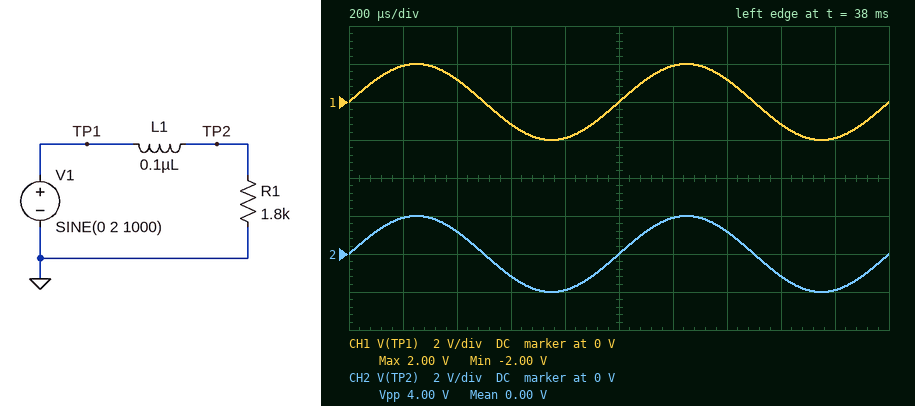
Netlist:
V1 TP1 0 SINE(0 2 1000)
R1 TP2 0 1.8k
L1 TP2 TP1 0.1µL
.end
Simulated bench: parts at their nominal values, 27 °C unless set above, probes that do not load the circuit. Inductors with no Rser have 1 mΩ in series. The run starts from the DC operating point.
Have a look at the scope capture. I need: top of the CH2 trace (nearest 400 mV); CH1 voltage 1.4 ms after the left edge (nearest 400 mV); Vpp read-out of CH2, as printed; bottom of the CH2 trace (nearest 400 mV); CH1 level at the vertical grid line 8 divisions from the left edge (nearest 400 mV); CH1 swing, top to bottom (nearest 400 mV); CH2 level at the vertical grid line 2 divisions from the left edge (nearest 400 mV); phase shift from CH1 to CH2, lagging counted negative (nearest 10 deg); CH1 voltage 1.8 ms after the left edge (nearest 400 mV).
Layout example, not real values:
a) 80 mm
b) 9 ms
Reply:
a) 2.0 V
b) 1.2 V
c) 4.00 V
d) -2.0 V
e) -1.2 V
f) 4.0 V
g) 1.2 V
h) 0 deg
i) -2.0 V
